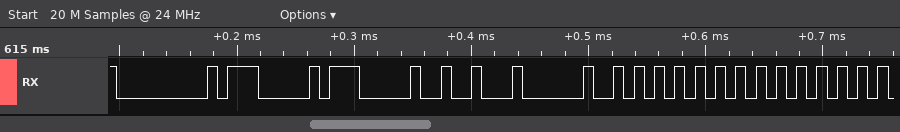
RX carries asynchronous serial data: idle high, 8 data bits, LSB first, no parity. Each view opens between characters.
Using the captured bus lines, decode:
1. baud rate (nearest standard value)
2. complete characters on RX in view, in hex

115200 baud
00, 07, 07, 12, 20, 55, 55
